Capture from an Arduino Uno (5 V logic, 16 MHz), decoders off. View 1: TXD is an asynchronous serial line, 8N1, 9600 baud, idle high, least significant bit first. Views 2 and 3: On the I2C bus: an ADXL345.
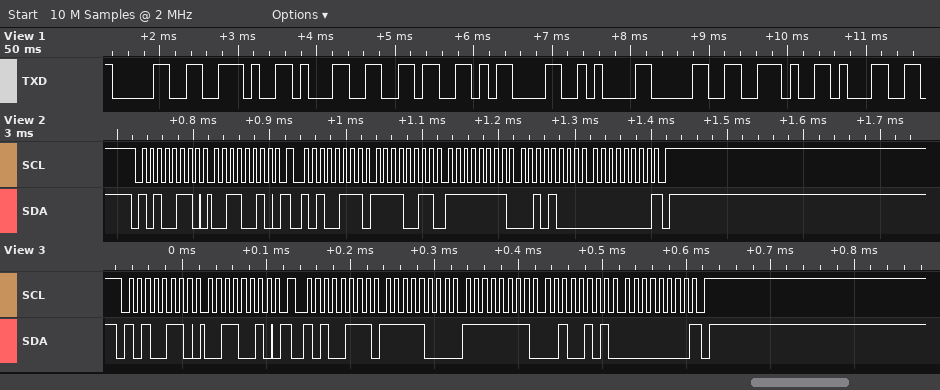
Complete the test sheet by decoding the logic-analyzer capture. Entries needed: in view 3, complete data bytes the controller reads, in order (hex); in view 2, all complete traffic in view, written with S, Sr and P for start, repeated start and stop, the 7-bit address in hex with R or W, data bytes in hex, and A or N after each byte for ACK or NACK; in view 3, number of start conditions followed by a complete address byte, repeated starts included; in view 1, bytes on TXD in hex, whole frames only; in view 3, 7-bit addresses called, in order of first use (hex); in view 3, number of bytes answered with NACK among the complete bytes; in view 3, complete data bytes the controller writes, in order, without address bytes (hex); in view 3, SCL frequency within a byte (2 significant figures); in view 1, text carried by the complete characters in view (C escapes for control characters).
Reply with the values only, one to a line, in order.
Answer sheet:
F8 FF 25 00
S 53W A 32 A Sr 53R A F3 A FF A 28 A 00 N P
2
30 2E 31 36 0D 0A 30 2E 31
0x53
1
32
100 kHz
"0.16\r\n0.1"
